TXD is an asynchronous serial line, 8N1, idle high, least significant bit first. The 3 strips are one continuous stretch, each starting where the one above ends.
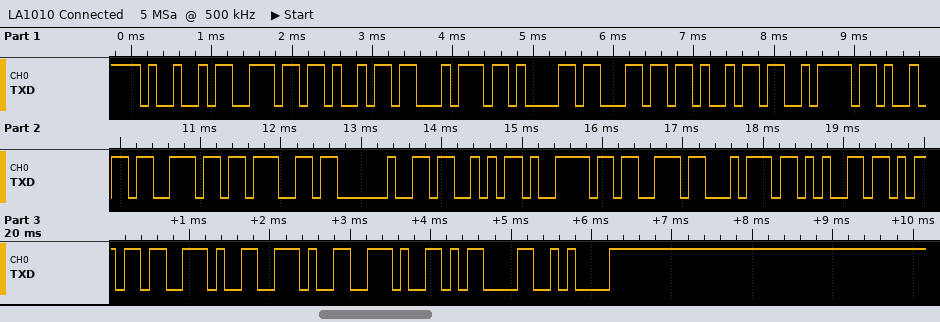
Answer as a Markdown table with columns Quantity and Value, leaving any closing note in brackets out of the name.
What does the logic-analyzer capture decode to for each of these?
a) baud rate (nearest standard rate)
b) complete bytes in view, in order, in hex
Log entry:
| Quantity | Value |
|---|---|
| baud rate | 9600 baud |
| complete bytes in view, in order, in hex | 49 6E 69 74 61 6C 69 7A 69 6E 67 20 53 79 73 74 65 6D 2E 2E 2E 0D 0A |
